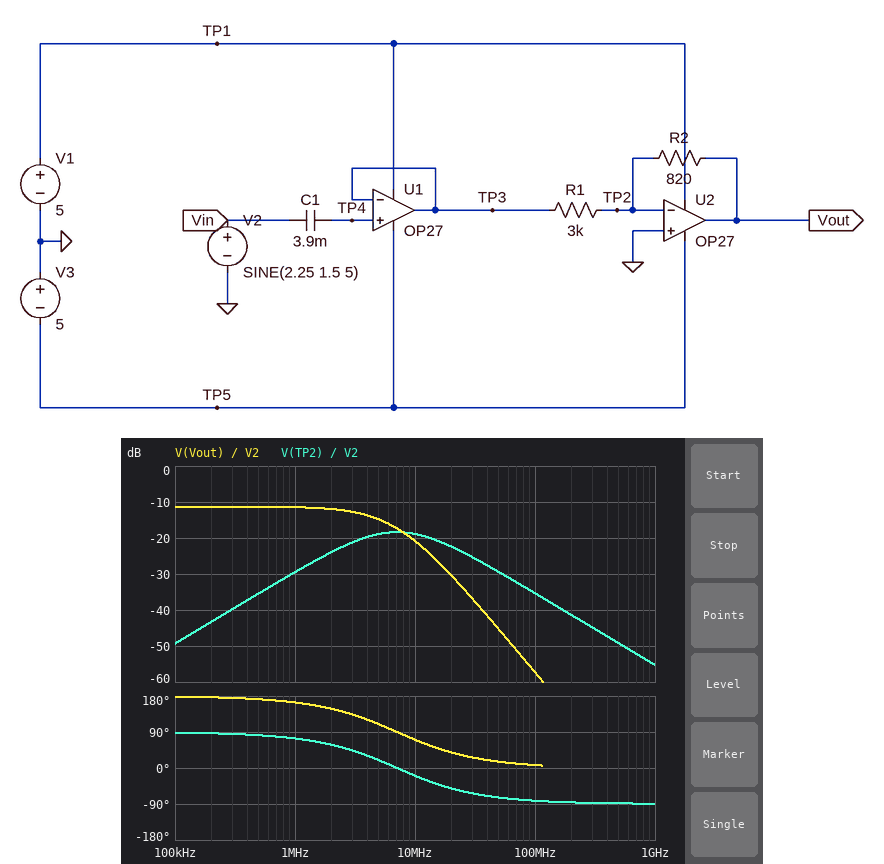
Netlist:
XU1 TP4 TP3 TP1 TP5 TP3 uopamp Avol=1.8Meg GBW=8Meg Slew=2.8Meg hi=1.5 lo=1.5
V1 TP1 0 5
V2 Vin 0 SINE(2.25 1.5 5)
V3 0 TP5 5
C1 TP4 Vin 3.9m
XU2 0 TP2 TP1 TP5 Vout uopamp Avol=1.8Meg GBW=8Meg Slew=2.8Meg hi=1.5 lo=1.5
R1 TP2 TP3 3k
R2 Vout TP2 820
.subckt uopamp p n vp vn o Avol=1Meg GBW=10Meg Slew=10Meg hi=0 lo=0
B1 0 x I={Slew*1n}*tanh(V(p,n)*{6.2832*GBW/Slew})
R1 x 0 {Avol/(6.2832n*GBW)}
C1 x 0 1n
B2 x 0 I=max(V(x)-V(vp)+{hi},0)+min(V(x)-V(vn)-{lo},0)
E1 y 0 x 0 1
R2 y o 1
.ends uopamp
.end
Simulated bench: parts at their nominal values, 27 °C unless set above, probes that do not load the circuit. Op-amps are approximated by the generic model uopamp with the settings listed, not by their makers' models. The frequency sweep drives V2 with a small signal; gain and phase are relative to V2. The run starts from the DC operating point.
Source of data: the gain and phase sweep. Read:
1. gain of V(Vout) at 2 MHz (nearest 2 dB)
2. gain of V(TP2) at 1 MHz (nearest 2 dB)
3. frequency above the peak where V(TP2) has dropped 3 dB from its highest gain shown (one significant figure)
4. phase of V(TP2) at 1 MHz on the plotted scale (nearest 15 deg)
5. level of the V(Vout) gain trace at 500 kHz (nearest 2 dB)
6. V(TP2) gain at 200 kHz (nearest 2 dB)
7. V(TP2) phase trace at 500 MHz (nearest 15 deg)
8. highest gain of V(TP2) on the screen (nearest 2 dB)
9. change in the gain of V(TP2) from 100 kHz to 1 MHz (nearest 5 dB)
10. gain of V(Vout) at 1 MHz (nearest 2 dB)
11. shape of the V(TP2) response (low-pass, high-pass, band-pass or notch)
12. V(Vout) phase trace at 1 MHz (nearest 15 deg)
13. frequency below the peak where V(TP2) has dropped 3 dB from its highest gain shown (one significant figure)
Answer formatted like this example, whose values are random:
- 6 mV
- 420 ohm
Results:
- -12 dB
- -30 dB
- 20 MHz
- 75 deg
- -12 dB
- -44 dB
- -90 deg
- -18 dB
- 20 dB
- -12 dB
- band-pass
- 165 deg
- 3 MHz
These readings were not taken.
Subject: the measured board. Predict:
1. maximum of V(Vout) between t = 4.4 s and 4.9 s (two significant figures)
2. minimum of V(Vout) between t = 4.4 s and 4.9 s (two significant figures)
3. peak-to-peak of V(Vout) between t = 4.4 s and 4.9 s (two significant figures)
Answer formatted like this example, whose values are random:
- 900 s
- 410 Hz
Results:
- 410 mV
- -410 mV
- 820 mV
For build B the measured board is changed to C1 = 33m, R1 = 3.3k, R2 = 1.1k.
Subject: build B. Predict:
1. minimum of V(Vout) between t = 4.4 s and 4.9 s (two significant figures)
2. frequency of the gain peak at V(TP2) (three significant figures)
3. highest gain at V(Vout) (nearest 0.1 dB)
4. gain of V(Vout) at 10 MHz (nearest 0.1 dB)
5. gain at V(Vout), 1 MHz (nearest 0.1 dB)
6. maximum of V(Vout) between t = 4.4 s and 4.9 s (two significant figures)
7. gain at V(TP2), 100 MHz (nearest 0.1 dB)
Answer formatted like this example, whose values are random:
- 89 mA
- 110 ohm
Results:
- -500 mV
- 6.93 MHz
- -9.5 dB
- -19.4 dB
- -9.7 dB
- 500 mV
- -34.0 dB
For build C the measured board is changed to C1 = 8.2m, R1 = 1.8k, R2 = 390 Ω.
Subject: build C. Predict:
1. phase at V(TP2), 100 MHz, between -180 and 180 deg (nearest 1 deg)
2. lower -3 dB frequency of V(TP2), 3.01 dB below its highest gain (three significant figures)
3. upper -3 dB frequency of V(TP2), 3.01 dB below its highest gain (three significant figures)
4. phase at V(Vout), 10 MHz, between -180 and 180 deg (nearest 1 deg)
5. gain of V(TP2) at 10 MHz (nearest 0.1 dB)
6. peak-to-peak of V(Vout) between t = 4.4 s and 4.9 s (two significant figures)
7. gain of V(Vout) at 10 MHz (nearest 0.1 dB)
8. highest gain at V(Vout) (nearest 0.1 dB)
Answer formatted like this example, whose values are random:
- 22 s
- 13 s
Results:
- -82 deg
- 2.99 MHz
- 17.6 MHz
- 72 deg
- -20.6 dB
- 650 mV
- -22.6 dB
- -13.3 dB
